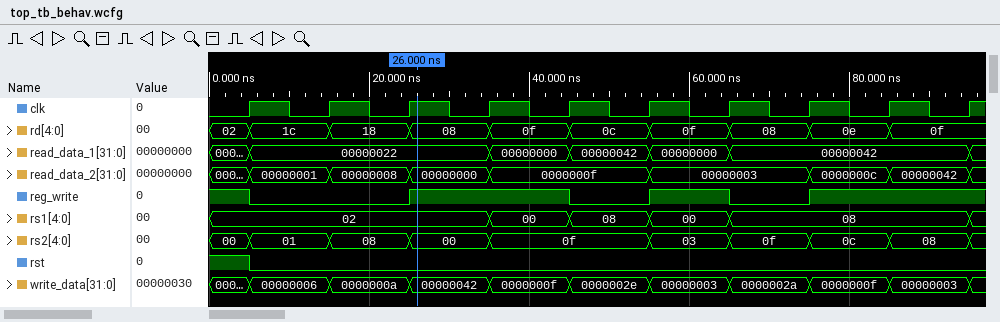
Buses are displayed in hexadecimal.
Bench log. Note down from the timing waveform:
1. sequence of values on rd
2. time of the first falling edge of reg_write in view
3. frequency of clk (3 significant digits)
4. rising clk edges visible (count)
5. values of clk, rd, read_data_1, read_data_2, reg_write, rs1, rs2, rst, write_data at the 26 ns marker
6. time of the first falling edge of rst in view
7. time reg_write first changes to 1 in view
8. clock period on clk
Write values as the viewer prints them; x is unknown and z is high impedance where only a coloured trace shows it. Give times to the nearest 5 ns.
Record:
02, 1c, 18, 08, 0f, 0c, 0f, 08, 0e, 0f
5 ns
100 MHz
10
clk=1, rd=08, read_data_1=00000022, read_data_2=00000000, reg_write=1, rs1=02, rs2=00, rst=0, write_data=00000042
5 ns
25 ns
10 ns
